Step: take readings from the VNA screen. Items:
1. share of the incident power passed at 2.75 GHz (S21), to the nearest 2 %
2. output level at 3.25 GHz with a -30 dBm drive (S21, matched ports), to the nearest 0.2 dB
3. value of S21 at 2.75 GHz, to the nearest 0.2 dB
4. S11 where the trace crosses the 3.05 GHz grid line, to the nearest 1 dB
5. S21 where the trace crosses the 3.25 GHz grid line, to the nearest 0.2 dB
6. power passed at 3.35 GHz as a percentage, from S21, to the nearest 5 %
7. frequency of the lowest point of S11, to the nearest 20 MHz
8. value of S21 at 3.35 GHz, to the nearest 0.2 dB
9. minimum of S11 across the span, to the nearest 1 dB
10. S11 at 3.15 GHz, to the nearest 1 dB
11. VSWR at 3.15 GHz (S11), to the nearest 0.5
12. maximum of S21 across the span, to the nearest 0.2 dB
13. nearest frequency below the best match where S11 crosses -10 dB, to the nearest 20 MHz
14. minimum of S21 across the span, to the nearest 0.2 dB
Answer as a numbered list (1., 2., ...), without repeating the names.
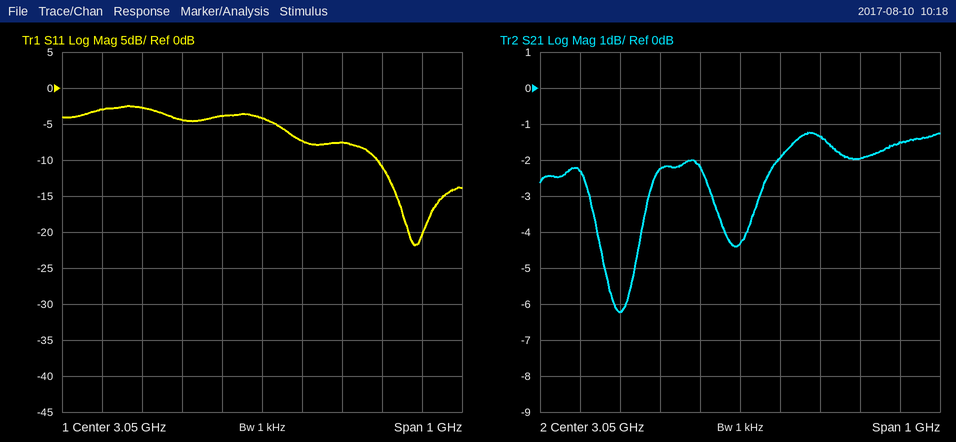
1. 24 %
2. -31.4 dBm
3. -6.2 dB
4. -4 dB
5. -1.4 dB
6. 65 %
7. 3.44 GHz
8. -2.0 dB
9. -22 dB
10. -7 dB
11. 2.5
12. -1.2 dB
13. 3.34 GHz
14. -6.2 dB
